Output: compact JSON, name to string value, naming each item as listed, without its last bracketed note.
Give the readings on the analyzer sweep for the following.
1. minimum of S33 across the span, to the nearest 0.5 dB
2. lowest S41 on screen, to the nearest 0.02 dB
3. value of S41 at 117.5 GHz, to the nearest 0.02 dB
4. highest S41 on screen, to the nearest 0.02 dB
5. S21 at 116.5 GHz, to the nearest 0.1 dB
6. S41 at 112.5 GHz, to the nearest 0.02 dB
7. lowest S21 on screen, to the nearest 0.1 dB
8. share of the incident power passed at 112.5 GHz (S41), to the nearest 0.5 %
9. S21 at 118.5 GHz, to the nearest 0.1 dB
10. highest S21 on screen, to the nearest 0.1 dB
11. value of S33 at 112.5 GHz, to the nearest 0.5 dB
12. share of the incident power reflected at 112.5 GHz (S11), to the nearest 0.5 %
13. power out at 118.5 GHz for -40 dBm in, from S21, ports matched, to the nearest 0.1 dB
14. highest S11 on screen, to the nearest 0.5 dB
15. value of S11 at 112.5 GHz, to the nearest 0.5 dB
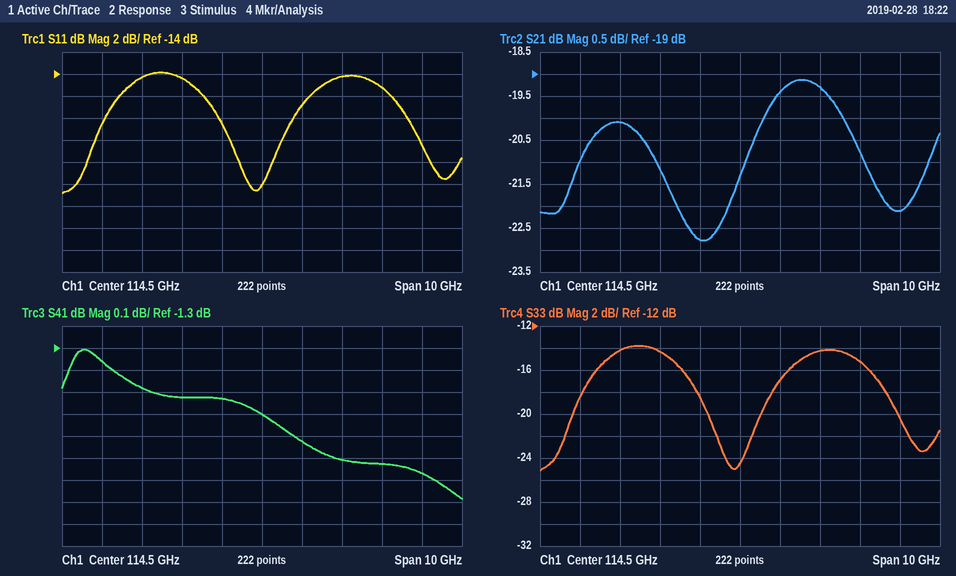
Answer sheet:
{"minimum of S33 across the span, to the nearest 0.5 dB": "-25.0 dB", "lowest S41 on screen, to the nearest 0.02 dB": "-1.98 dB", "value of S41 at 117.5 GHz, to the nearest 0.02 dB": "-1.82 dB", "highest S41 on screen, to the nearest 0.02 dB": "-1.30 dB", "S21 at 116.5 GHz, to the nearest 0.1 dB": "-19.3 dB", "S41 at 112.5 GHz, to the nearest 0.02 dB": "-1.52 dB", "lowest S21 on screen, to the nearest 0.1 dB": "-22.8 dB", "share of the incident power passed at 112.5 GHz (S41), to the nearest 0.5 %": "70.5 %", "S21 at 118.5 GHz, to the nearest 0.1 dB": "-22.1 dB", "highest S21 on screen, to the nearest 0.1 dB": "-19.1 dB", "value of S33 at 112.5 GHz, to the nearest 0.5 dB": "-14.5 dB", "share of the incident power reflected at 112.5 GHz (S11), to the nearest 0.5 %": "3.5 %", "power out at 118.5 GHz for -40 dBm in, from S21, ports matched, to the nearest 0.1 dB": "-62.1 dBm", "highest S11 on screen, to the nearest 0.5 dB": "-14.0 dB", "value of S11 at 112.5 GHz, to the nearest 0.5 dB": "-14.5 dB"}
